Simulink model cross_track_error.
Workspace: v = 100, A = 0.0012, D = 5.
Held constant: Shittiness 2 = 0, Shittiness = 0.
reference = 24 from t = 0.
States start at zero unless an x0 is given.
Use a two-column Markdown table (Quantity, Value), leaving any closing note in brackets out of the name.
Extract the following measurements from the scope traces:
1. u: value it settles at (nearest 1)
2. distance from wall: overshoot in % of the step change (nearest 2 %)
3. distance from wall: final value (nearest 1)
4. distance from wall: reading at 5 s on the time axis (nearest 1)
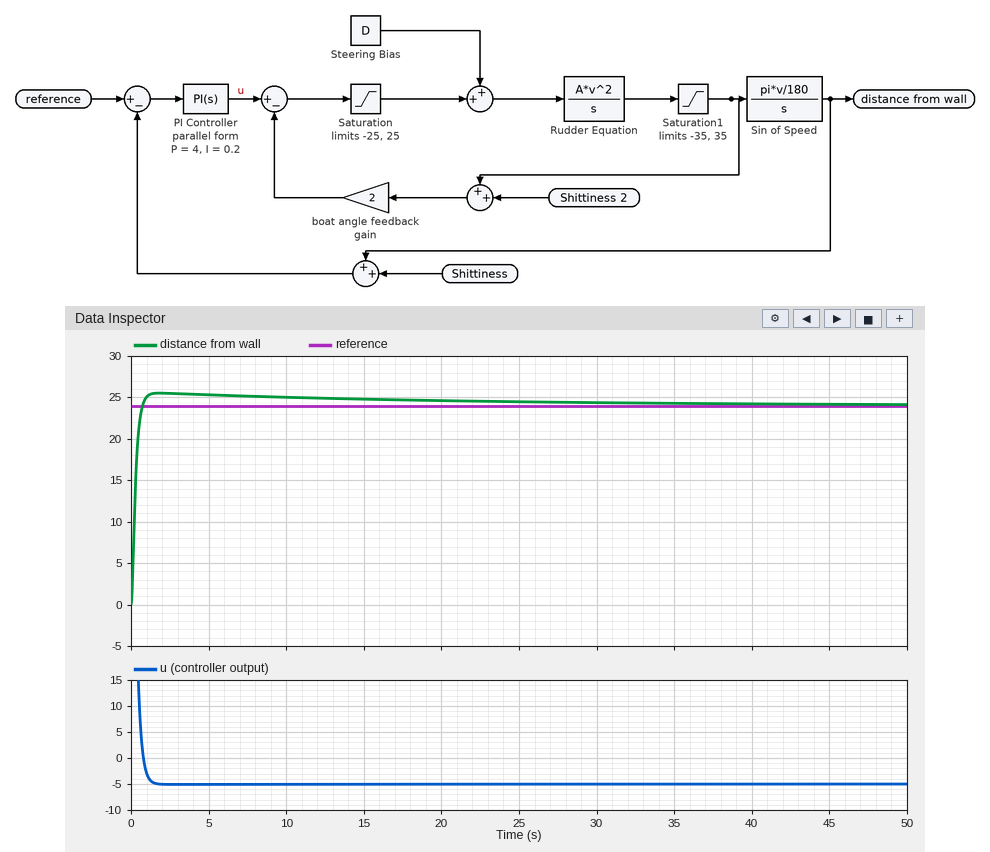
| Quantity | Value |
|---|---|
| u: value it settles at | -5 |
| distance from wall: overshoot in % of the step change | 6 % |
| distance from wall: final value | 24 |
| distance from wall: reading at 5 s on the time axis | 25 |
